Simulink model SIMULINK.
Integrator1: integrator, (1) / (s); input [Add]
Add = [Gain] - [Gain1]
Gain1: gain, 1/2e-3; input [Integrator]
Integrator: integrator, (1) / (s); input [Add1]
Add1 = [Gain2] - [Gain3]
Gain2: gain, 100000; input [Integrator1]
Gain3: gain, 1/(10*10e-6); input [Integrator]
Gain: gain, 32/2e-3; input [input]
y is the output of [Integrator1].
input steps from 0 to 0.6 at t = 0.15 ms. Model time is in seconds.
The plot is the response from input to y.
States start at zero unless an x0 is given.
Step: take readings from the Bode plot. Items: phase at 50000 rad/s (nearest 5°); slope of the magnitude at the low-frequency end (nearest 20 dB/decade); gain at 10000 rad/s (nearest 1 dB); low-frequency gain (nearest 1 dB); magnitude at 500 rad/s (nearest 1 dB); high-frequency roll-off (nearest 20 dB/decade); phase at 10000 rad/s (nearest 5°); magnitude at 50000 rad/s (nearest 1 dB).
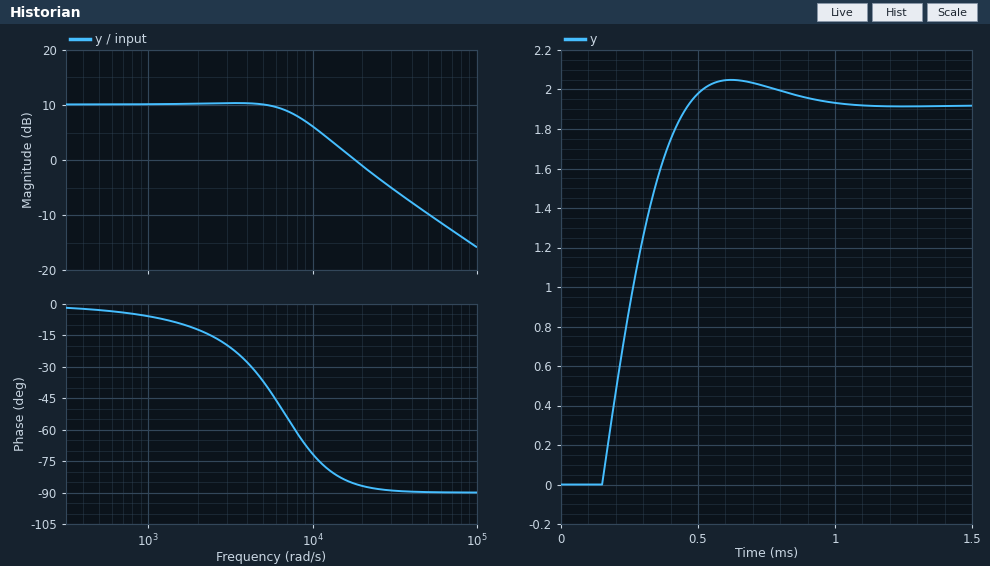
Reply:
-90°
0 dB/decade
6 dB
10 dB
10 dB
-20 dB/decade
-70°
-10 dB
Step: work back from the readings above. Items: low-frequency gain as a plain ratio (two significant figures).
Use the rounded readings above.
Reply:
3.2
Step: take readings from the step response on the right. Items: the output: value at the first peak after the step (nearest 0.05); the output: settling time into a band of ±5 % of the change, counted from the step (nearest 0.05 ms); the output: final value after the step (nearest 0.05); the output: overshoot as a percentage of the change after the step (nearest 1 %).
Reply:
2.05
0.60 ms
1.90
7 %
